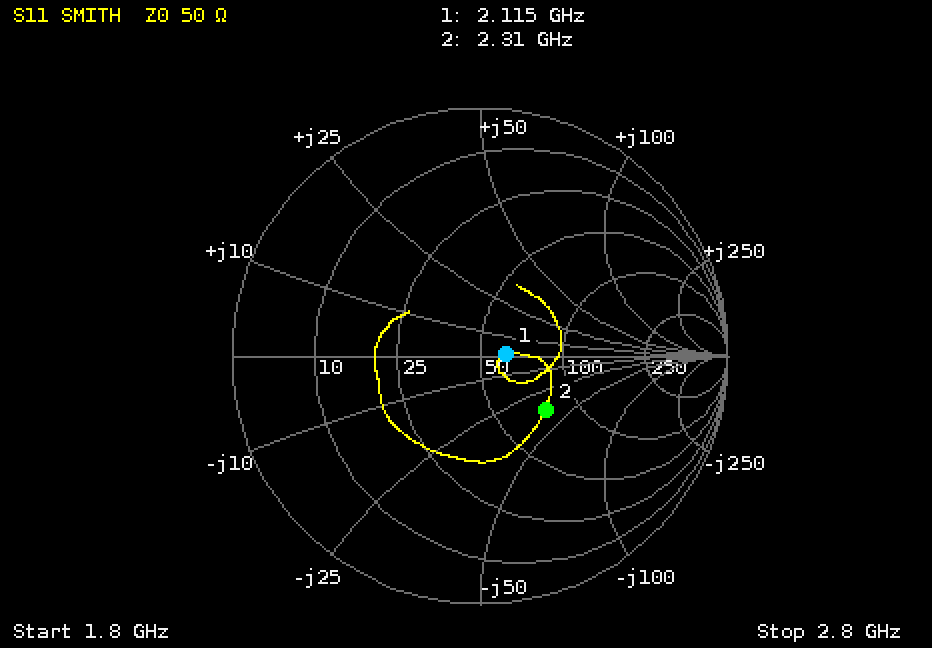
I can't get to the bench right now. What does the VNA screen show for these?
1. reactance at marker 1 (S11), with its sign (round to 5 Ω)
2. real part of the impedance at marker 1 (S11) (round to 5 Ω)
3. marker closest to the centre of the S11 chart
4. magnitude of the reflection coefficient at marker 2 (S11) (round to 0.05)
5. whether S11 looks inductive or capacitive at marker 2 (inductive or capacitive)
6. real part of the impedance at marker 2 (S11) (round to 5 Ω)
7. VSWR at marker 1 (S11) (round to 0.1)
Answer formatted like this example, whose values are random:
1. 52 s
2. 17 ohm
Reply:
1. 0 Ω
2. 60 Ω
3. marker 1
4. 0.35
5. capacitive
6. 75 Ω
7. 1.2
